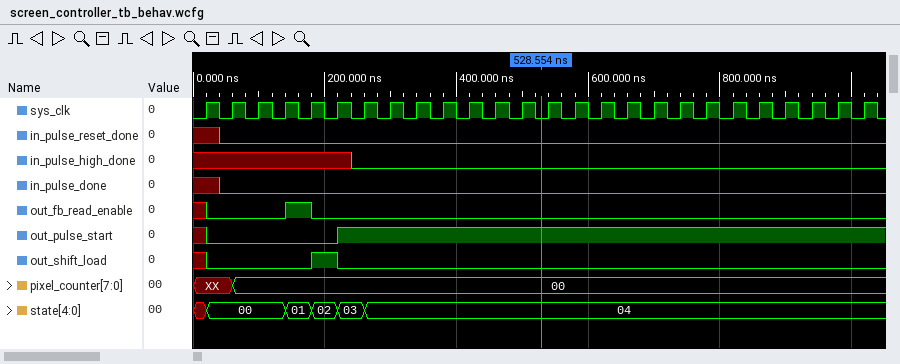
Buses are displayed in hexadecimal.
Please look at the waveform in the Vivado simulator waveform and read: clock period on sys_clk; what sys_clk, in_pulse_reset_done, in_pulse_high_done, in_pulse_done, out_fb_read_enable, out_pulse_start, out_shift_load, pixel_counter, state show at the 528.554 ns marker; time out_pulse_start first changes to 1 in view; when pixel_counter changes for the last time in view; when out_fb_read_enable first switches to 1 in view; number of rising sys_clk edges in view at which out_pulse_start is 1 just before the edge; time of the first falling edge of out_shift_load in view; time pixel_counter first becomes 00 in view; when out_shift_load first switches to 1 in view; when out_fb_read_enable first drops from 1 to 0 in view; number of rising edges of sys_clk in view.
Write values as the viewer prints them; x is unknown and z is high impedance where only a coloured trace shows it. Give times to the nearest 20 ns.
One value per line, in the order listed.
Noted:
40 ns
sys_clk=0, in_pulse_reset_done=0, in_pulse_high_done=0, in_pulse_done=0, out_fb_read_enable=0, out_pulse_start=1, out_shift_load=0, pixel_counter=00, state=04
220 ns
60 ns
140 ns
20
220 ns
60 ns
180 ns
180 ns
26
